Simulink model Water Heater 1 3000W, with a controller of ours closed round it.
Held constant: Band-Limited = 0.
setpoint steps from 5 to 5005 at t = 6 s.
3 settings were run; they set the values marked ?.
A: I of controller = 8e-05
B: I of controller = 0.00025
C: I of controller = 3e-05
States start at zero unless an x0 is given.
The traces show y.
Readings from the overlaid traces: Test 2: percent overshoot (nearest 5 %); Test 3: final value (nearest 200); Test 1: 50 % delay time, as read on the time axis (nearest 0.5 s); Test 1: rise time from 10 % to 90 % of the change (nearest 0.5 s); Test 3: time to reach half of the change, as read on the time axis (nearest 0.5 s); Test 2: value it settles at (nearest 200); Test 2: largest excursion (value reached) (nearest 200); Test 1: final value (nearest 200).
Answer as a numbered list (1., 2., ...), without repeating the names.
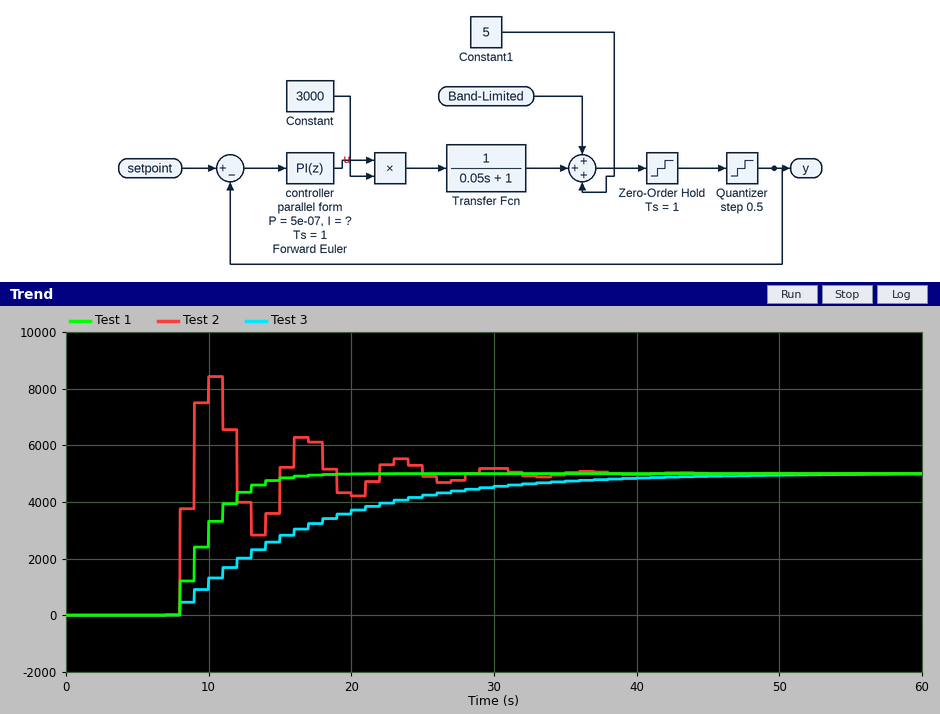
1. 70 %
2. 5000
3. 10.0 s
4. 5.0 s
5. 14.0 s
6. 5000
7. 8400
8. 5000
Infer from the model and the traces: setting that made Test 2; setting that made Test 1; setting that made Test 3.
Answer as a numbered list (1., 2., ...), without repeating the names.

1. B
2. A
3. C
